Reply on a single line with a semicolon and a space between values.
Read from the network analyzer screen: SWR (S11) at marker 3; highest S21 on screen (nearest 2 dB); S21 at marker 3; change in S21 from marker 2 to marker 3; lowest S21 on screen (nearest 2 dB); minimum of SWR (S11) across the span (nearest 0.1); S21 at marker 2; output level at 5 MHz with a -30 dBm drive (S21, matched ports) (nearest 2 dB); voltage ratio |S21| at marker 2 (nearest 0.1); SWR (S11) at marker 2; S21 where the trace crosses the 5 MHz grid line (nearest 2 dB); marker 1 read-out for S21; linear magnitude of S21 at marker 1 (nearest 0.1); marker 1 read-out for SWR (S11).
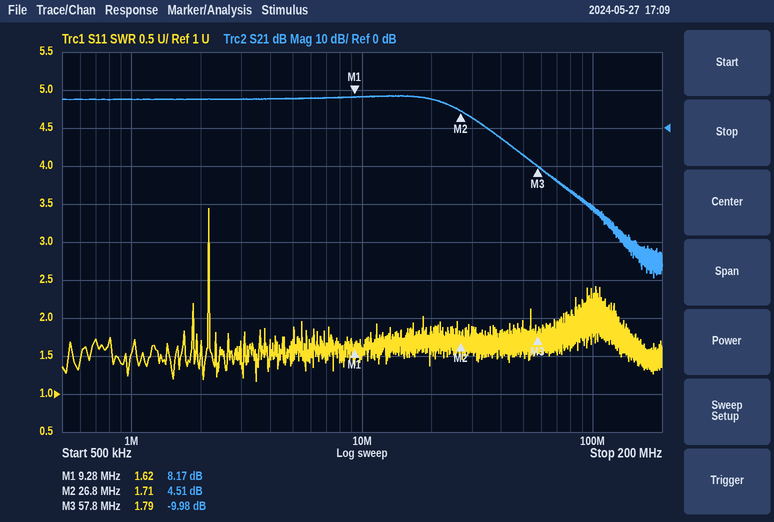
1.79; 8 dB; -9.98 dB; -14.49 dB; -40 dB; 1.2; 4.51 dB; -22 dBm; 1.7; 1.71; 8 dB; 8.17 dB; 2.6; 1.62
